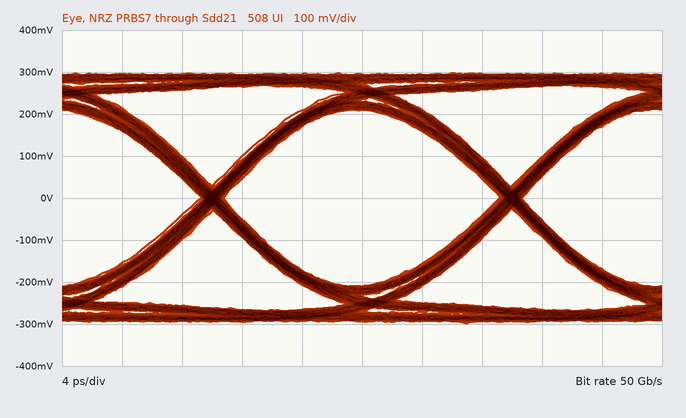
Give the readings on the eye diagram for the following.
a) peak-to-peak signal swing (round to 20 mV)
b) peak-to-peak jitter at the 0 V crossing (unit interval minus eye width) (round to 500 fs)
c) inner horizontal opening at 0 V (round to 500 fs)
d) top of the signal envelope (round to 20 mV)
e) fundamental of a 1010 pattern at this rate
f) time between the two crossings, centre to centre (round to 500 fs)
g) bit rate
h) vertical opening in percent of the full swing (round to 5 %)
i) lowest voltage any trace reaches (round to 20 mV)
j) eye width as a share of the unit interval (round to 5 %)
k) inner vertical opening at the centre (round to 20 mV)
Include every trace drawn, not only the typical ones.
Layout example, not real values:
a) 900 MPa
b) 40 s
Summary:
a) 600 mV
b) 1.5 ps
c) 18.5 ps
d) 300 mV
e) 25 GHz
f) 20.0 ps
g) 50 Gb/s
h) 70 %
i) -300 mV
j) 90 %
k) 420 mV
